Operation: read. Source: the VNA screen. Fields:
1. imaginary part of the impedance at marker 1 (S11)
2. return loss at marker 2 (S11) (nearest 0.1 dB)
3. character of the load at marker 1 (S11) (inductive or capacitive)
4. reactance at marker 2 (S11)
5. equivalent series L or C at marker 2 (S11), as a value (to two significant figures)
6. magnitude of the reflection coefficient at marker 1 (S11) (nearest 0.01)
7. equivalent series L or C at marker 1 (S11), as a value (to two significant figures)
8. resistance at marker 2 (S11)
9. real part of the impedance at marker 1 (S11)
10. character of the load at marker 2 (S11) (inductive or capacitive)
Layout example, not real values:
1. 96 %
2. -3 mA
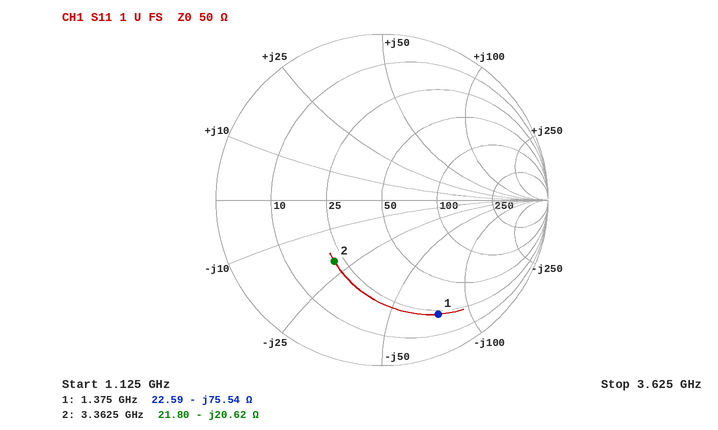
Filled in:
1. -75.54 Ω
2. 6.6 dB
3. capacitive
4. -20.62 Ω
5. 2.3 pF
6. 0.77
7. 1.5 pF
8. 21.80 Ω
9. 22.59 Ω
10. capacitive
